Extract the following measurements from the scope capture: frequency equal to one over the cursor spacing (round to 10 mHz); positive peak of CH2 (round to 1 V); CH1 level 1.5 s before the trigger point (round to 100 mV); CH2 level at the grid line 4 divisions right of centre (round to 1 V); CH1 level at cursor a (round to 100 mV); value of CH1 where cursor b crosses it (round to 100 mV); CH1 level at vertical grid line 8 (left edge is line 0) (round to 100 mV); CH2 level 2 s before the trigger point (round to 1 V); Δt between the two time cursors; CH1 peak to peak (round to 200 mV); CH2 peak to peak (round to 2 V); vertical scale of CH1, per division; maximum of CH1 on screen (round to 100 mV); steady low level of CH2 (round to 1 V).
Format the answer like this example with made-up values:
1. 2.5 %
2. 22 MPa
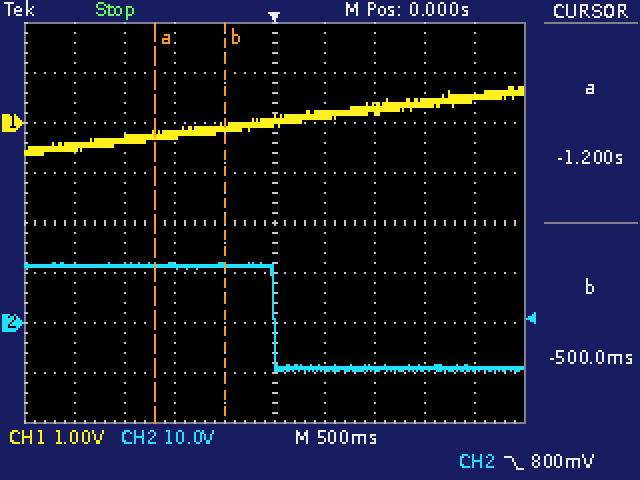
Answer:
1. 1.43 Hz
2. 12 V
3. -300 mV
4. -9 V
5. -200 mV
6. -100 mV
7. 400 mV
8. 11 V
9. 700 ms
10. 1.4 V
11. 22 V
12. 1 V
13. 700 mV
14. -9 V
